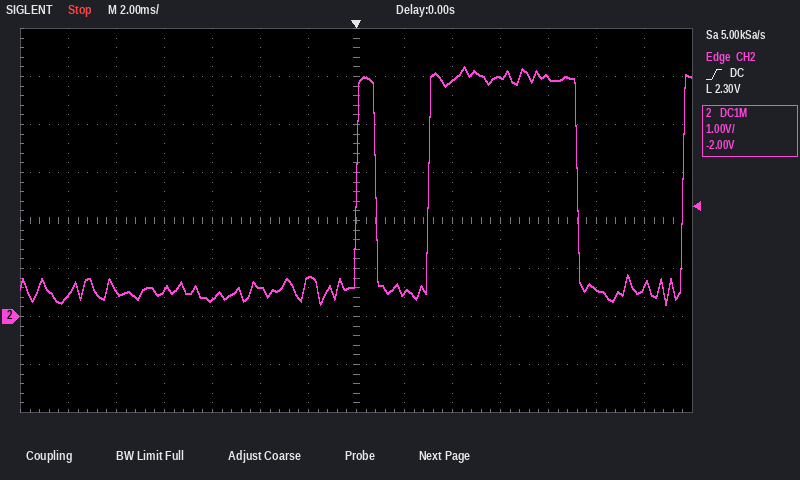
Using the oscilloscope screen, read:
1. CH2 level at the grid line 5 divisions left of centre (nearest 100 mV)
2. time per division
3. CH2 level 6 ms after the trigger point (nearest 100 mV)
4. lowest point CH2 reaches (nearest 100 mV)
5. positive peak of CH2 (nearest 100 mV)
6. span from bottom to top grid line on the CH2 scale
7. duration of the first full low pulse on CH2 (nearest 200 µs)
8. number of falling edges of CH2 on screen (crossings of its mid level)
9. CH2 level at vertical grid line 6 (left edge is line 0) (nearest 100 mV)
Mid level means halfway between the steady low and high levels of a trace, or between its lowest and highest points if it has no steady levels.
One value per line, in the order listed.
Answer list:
500 mV
2 ms
5.0 V
200 mV
5.2 V
8 V
2.2 ms
2
800 mV
